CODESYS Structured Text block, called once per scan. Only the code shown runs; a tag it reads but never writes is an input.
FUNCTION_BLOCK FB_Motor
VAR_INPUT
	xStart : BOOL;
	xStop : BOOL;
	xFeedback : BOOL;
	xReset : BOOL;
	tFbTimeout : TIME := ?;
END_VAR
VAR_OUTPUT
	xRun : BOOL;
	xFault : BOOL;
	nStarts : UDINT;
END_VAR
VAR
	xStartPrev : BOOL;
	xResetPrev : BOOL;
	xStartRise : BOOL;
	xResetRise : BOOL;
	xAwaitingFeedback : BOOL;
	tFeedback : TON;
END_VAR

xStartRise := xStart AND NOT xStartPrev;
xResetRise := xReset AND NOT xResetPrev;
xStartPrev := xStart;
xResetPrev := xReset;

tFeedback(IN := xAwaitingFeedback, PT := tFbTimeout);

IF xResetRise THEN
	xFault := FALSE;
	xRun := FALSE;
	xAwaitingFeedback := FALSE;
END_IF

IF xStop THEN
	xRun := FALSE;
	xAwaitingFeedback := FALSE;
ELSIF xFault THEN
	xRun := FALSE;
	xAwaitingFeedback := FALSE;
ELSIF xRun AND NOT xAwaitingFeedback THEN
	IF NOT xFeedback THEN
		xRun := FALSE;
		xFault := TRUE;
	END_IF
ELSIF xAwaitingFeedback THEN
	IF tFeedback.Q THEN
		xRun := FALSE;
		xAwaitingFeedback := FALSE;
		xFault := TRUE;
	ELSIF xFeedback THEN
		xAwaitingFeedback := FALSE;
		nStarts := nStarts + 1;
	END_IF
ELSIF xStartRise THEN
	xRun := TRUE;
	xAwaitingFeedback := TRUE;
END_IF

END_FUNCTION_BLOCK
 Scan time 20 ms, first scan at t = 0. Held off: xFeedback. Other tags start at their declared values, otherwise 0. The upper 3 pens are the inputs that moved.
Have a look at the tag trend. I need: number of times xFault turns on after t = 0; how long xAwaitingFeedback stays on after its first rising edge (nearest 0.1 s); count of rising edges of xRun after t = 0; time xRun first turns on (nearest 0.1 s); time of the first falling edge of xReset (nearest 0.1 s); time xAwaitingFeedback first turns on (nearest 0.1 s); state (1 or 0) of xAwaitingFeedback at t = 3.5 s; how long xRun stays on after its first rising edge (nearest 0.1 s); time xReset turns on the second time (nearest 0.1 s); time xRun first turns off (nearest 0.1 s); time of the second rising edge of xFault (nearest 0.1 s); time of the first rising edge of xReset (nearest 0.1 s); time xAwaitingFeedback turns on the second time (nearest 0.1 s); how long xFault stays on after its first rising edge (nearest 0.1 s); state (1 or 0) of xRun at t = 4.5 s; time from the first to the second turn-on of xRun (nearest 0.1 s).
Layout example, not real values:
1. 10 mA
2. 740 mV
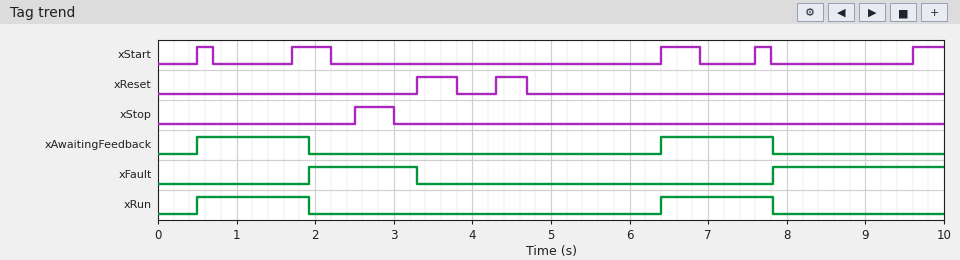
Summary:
1. 2
2. 1.4 s
3. 2
4. 0.5 s
5. 3.8 s
6. 0.5 s
7. 0
8. 1.4 s
9. 4.3 s
10. 1.9 s
11. 7.8 s
12. 3.3 s
13. 6.4 s
14. 1.4 s
15. 0
16. 5.9 s
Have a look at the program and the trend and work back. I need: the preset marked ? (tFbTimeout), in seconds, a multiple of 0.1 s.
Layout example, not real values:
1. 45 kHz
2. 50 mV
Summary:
1. 1.4 s
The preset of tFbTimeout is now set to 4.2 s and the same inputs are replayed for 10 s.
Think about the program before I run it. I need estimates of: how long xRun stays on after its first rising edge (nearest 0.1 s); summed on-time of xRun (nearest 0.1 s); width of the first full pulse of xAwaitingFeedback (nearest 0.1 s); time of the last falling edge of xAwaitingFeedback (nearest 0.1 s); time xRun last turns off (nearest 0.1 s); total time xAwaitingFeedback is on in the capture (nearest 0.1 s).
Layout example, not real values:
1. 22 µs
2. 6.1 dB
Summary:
1. 2.0 s
2. 5.6 s
3. 2.0 s
4. 2.5 s
5. 2.5 s
6. 5.6 s
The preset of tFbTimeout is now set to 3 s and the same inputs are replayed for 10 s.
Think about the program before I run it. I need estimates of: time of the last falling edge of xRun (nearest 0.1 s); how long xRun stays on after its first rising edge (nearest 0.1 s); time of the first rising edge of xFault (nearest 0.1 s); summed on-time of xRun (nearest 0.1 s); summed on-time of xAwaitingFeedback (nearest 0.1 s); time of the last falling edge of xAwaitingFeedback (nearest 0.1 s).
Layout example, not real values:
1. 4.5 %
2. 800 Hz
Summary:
1. 9.4 s
2. 2.0 s
3. 9.4 s
4. 5.0 s
5. 5.0 s
6. 9.4 s
